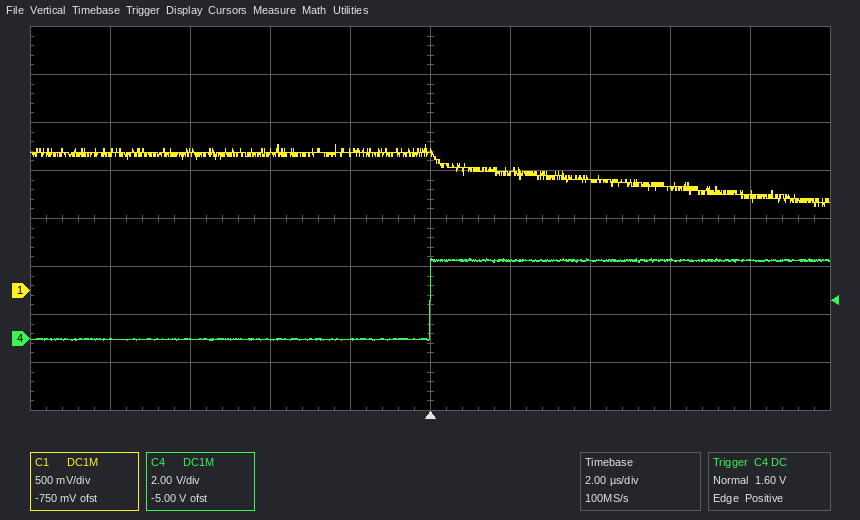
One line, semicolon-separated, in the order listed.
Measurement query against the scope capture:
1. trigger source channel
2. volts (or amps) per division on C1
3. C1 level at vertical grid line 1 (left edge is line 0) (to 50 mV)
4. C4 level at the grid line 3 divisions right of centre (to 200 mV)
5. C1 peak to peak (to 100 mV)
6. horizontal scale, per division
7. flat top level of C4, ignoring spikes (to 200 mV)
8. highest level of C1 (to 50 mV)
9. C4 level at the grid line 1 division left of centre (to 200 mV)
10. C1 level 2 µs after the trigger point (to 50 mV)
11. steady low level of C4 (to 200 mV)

C4; 500 mV; 1.45 V; 3.2 V; 600 mV; 2 µs; 3.2 V; 1.50 V; 0.0 V; 1.25 V; 0.0 V
